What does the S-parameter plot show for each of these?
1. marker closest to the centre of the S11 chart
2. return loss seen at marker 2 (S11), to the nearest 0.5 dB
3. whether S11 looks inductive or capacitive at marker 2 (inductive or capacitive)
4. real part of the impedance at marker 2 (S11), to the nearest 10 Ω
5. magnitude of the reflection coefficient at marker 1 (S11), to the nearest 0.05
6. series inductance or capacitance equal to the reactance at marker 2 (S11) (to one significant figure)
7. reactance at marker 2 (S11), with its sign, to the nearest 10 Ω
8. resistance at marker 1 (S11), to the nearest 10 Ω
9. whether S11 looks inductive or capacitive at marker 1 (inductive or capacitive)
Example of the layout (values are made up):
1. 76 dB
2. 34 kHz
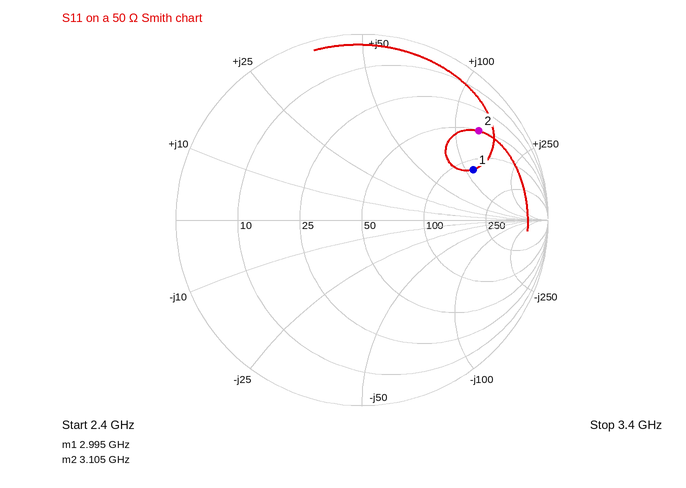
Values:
1. marker 1
2. 2.0 dB
3. inductive
4. 50 Ω
5. 0.65
6. 7 nH
7. +130 Ω
8. 120 Ω
9. inductive
